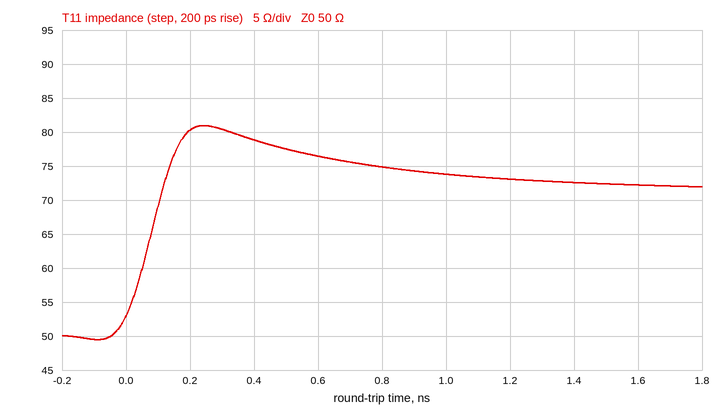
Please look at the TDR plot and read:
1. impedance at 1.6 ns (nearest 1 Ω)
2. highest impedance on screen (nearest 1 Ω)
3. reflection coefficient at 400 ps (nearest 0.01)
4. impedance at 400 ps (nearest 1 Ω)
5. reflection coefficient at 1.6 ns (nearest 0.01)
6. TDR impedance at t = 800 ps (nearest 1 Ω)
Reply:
72 Ω
81 Ω
+0.22
79 Ω
+0.18
75 Ω
